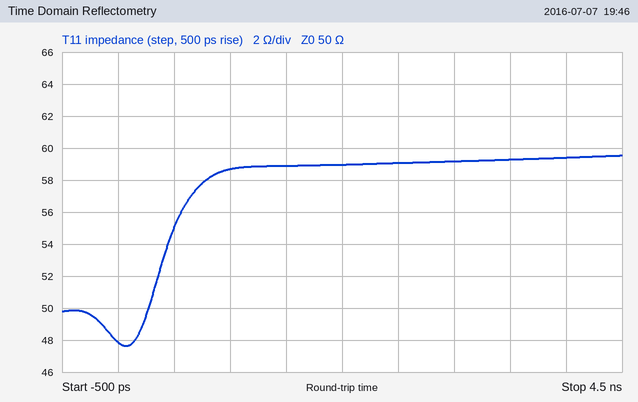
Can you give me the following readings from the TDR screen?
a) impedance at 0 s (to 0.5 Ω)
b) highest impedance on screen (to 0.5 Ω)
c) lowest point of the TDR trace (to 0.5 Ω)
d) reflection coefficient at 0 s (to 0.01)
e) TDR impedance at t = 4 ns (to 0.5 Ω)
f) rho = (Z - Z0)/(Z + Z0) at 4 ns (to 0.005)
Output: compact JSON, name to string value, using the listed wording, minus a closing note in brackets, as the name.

{"impedance at 0 s": "48.0 Ω", "highest impedance on screen": "59.5 Ω", "lowest point of the TDR trace": "47.5 Ω", "reflection coefficient at 0 s": "-0.02", "TDR impedance at t = 4 ns": "59.5 Ω", "rho = (Z - Z0)/(Z + Z0) at 4 ns": "+0.085"}
